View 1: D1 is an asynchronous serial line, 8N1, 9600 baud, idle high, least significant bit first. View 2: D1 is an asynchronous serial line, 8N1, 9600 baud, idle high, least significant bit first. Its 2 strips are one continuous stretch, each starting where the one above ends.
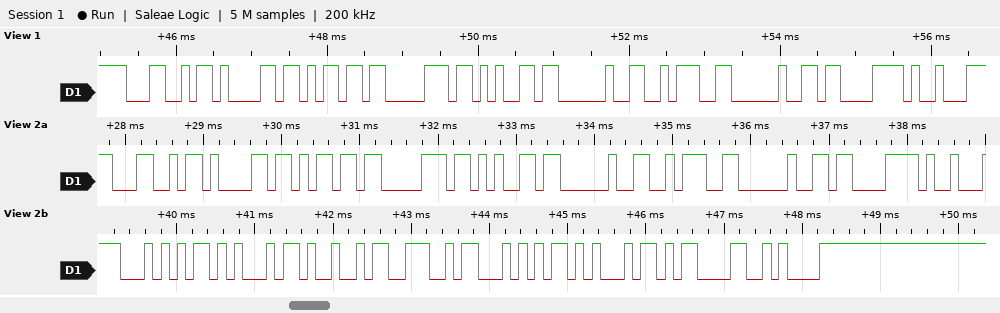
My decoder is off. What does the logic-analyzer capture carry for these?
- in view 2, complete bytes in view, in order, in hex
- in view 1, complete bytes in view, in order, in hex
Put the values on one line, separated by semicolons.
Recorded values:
0x4C 0x61 0x6D 0x70 0x65 0x20 0x3A 0x20 0xC3 0x89 0x54 0x45 0x49 0x4E 0x54 0x45 0x0D 0x0A; 4C 61 6D 70 65 20 3A 20 C3 89
